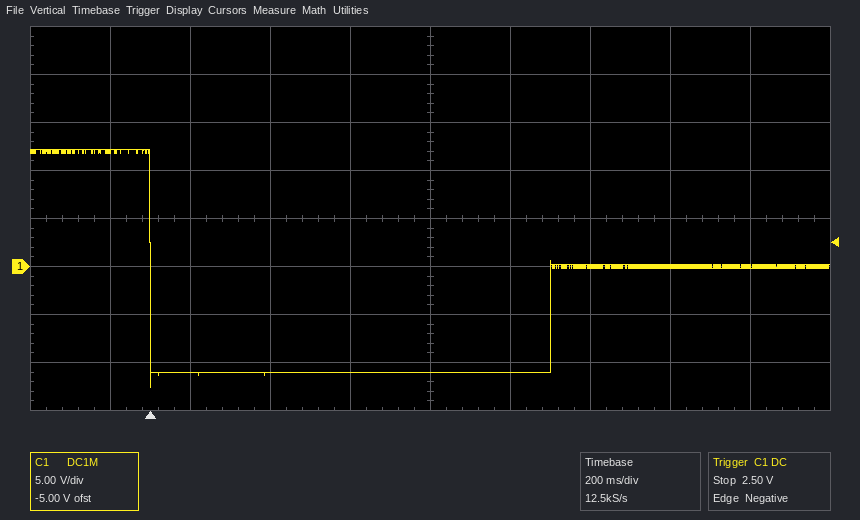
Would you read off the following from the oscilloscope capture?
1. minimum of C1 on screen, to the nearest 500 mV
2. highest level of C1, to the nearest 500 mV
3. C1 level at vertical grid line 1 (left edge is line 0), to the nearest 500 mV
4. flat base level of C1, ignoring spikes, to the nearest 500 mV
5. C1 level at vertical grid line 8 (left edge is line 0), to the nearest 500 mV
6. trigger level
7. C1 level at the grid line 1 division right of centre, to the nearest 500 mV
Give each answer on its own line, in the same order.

-12.5 V
12.0 V
12.0 V
-11.0 V
0.0 V
2.50 V
-11.0 V
